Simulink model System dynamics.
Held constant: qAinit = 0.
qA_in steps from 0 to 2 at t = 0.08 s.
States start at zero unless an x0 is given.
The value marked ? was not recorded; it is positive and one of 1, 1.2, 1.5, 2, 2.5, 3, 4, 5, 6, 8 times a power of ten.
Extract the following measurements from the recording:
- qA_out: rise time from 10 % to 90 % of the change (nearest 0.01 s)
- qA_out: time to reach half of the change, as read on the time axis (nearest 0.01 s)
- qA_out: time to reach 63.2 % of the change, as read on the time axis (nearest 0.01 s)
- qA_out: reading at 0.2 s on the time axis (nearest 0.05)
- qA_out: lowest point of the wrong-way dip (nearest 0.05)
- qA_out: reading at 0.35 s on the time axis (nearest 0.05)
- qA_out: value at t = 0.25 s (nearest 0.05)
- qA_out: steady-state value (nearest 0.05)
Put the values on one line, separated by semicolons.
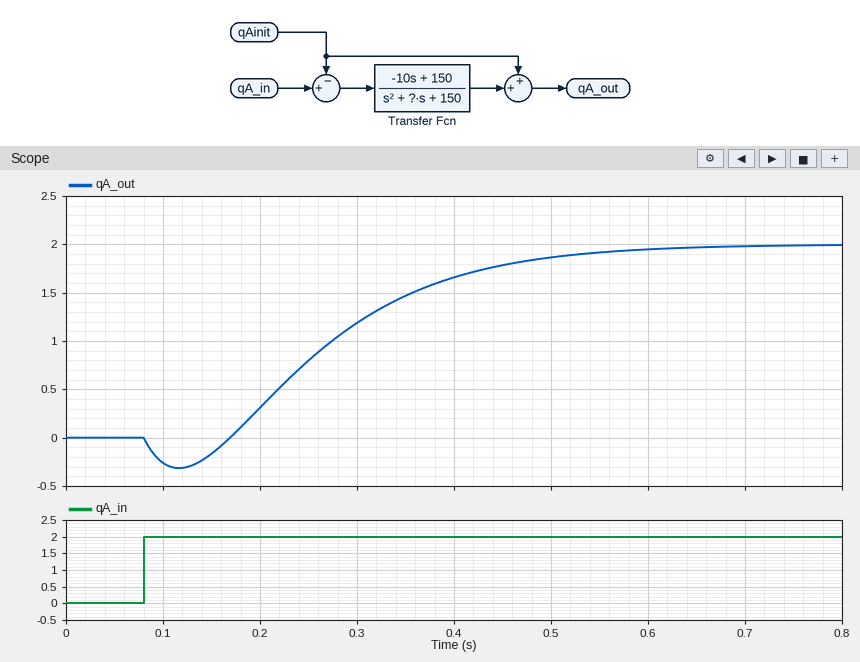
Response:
0.27 s; 0.27 s; 0.31 s; 0.30; -0.30; 1.45; 0.80; 2.00
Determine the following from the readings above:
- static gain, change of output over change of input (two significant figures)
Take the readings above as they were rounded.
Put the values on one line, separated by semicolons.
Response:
1.0
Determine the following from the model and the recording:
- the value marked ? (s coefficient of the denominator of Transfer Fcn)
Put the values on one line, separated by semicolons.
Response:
25
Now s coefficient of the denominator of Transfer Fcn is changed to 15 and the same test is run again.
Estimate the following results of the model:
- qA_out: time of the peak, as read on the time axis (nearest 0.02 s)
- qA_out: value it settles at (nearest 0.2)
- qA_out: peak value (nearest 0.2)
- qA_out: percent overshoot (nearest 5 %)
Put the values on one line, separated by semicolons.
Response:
0.44 s; 2.0; 2.2; 10 %
